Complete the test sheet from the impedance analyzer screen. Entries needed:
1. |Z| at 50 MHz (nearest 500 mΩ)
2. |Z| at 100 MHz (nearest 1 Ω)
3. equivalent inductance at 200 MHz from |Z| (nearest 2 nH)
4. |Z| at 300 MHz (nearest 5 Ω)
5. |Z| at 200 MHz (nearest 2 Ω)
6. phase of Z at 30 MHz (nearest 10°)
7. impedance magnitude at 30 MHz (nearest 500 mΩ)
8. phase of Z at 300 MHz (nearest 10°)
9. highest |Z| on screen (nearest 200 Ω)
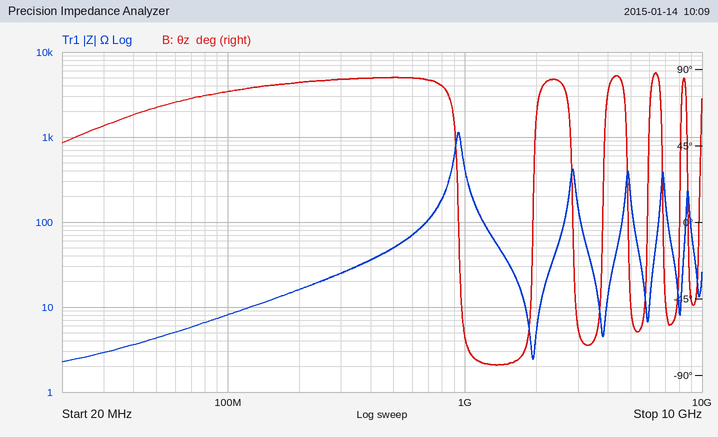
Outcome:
4.5 Ω
8 Ω
12 nH
25 Ω
16 Ω
60°
3.0 Ω
80°
1.2 kΩ
